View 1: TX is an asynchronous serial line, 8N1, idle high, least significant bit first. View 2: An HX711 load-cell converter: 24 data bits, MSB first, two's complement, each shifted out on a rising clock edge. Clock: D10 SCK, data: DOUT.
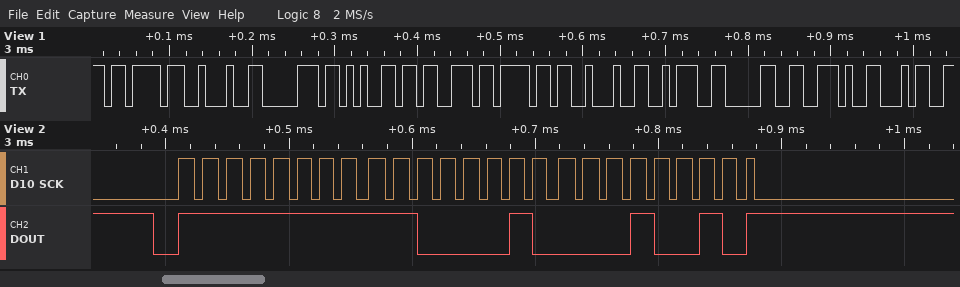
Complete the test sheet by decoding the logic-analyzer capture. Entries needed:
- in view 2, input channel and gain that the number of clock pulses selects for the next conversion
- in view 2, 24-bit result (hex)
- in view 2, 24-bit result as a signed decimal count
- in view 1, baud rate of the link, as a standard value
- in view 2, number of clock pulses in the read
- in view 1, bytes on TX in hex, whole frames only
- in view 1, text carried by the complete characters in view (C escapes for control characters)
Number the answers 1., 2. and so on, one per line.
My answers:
1. channel A, gain 128
2. 0xFFC212
3. -15854
4. 115200 baud
5. 25
6. 7B 22 70 65 73 6F 22 3A 30 2E 34
7. "{\"peso\":0.4"
